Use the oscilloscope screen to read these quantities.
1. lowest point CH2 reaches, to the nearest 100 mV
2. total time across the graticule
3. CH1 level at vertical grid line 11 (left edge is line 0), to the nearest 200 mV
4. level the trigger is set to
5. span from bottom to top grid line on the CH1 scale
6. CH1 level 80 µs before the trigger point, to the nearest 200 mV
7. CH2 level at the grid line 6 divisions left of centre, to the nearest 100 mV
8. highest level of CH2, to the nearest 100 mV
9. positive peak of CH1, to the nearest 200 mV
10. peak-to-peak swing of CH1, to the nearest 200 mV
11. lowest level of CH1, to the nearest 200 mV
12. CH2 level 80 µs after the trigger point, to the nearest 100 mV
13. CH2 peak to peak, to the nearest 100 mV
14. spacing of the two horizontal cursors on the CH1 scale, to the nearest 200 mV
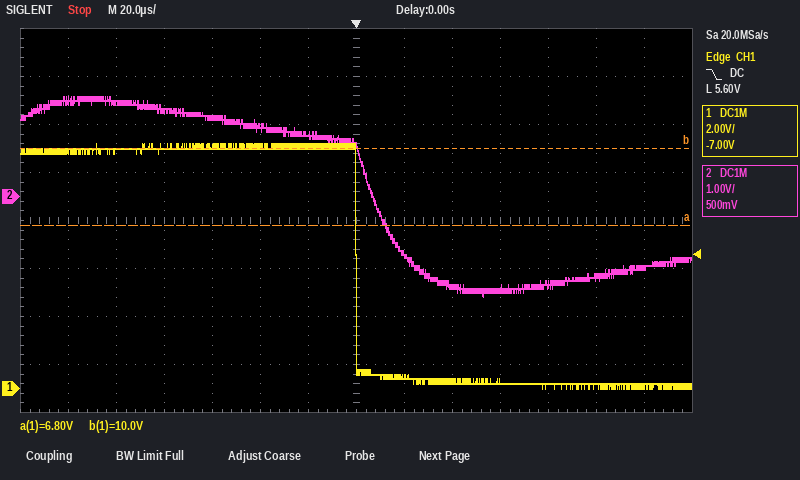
-2.1 V
280 µs
200 mV
5.60 V
16 V
10.0 V
2.0 V
2.1 V
10.2 V
10.2 V
0.0 V
-1.8 V
4.2 V
3.2 V
